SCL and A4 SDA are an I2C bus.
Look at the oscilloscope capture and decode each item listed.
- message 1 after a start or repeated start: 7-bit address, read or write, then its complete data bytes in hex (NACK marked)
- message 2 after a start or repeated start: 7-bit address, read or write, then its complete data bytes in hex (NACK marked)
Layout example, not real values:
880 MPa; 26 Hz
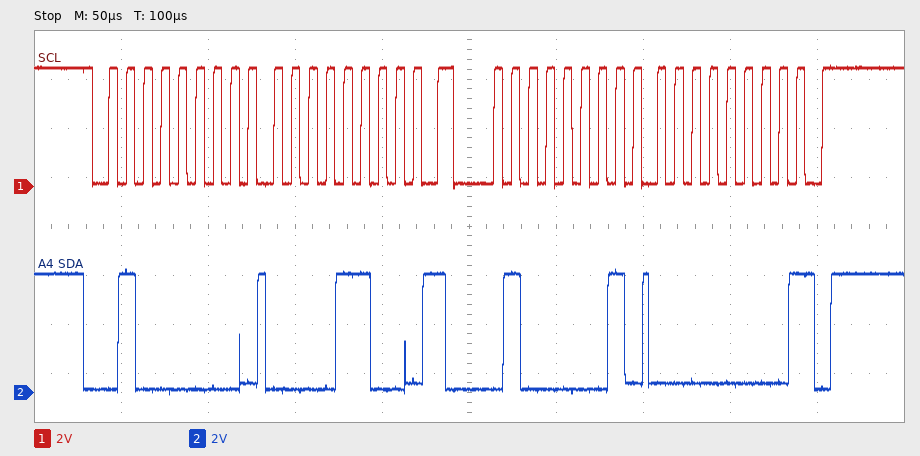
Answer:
0x20 write: 0C; 0x20 read: 00 NACK
